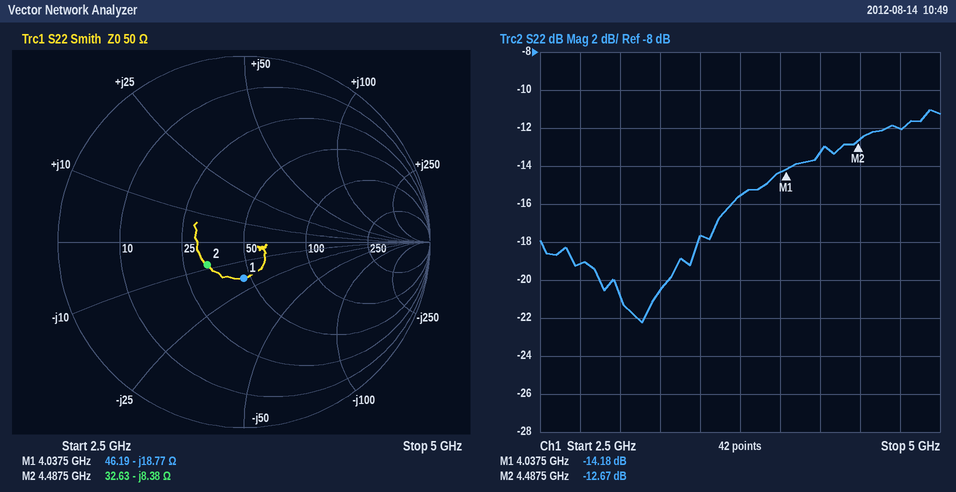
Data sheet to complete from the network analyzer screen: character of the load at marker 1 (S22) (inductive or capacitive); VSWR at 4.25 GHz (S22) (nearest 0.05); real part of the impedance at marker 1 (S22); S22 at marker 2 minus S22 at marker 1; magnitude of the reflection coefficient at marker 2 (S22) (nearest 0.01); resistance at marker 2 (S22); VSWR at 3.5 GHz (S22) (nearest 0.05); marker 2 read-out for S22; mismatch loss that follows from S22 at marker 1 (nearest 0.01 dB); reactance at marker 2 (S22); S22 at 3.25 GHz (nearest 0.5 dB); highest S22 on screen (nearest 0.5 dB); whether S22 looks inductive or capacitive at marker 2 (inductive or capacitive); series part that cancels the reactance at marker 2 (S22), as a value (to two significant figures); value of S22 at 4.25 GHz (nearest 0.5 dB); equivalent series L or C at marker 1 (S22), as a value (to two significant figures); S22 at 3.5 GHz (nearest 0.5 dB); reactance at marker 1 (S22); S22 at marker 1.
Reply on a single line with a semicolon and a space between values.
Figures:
capacitive; 1.55; 46.19 Ω; 1.51 dB; 0.23; 32.63 Ω; 1.30; -12.67 dB; 0.17 dB; -8.38 Ω; -20.5 dB; -11.0 dB; capacitive; 300 pH; -13.5 dB; 2.1 pF; -17.5 dB; -18.77 Ω; -14.18 dB
